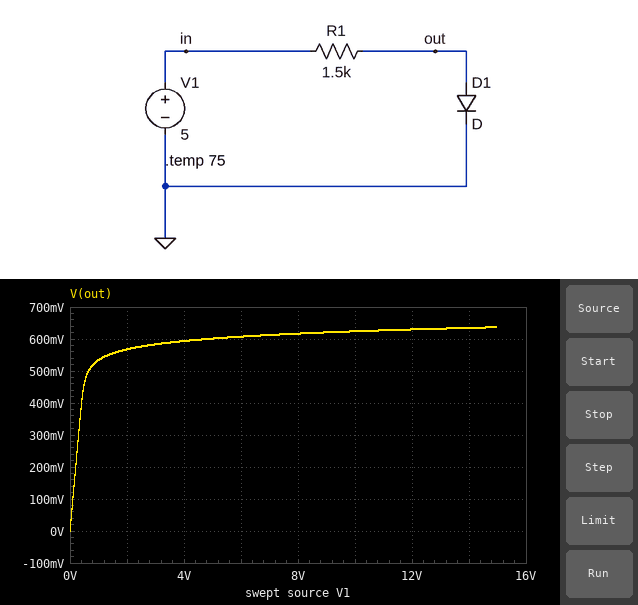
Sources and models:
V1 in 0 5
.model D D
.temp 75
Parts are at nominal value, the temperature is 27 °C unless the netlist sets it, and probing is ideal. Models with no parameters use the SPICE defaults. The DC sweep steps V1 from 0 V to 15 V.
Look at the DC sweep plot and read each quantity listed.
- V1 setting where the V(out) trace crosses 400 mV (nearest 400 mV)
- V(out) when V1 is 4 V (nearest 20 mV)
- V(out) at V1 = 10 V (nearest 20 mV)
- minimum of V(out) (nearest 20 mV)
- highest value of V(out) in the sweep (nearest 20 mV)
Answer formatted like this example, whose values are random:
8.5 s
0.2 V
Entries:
400 mV
600 mV
620 mV
0 V
640 mV
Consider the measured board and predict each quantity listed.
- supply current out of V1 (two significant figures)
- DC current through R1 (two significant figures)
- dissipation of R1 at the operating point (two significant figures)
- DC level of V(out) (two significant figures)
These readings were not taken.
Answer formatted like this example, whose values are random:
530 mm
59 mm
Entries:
2.9 mA
2.9 mA
13 mW
600 mV
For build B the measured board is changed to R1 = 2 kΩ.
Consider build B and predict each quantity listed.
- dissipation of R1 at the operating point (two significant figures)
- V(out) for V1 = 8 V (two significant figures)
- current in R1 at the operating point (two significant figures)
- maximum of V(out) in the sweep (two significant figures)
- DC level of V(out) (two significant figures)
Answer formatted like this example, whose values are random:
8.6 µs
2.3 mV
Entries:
9.7 mW
610 mV
2.2 mA
630 mV
590 mV
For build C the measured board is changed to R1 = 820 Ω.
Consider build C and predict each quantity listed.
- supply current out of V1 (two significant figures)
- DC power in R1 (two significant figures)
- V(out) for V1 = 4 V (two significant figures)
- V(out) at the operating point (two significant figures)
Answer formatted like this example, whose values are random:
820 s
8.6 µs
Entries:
5.3 mA
23 mW
610 mV
620 mV
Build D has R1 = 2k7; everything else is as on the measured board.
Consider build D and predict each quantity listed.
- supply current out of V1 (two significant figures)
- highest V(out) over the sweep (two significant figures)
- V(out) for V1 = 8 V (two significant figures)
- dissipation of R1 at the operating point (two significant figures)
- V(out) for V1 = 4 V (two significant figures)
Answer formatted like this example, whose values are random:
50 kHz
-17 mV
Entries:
1.6 mA
620 mV
600 mV
7.2 mW
580 mV
